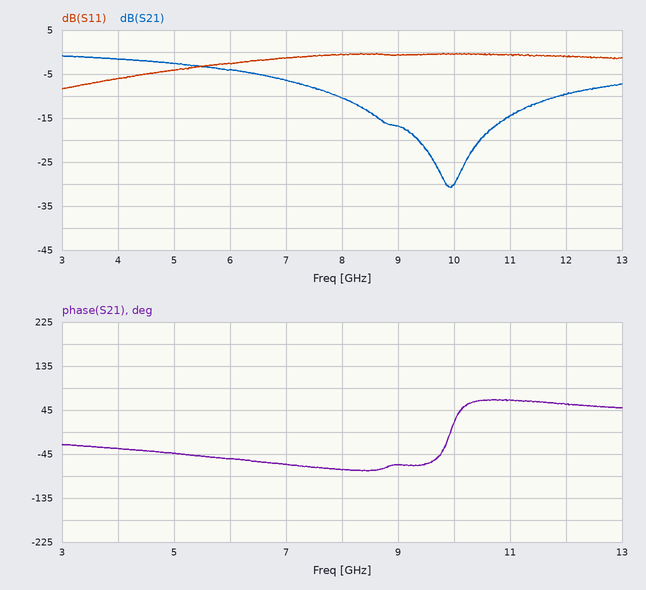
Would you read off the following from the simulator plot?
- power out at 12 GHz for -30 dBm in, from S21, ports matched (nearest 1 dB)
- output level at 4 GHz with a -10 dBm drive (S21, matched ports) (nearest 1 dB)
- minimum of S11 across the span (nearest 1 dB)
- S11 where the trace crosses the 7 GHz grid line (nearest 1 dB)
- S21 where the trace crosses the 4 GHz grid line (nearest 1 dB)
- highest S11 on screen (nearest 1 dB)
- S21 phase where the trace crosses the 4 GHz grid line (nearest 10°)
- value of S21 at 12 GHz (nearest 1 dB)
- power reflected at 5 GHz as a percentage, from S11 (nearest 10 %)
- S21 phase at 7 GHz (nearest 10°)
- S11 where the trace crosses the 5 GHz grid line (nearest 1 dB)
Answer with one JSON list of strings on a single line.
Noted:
["-40 dBm", "-12 dBm", "-8 dB", "-1 dB", "-2 dB", "0 dB", "-30°", "-10 dB", "40 %", "-70°", "-4 dB"]
